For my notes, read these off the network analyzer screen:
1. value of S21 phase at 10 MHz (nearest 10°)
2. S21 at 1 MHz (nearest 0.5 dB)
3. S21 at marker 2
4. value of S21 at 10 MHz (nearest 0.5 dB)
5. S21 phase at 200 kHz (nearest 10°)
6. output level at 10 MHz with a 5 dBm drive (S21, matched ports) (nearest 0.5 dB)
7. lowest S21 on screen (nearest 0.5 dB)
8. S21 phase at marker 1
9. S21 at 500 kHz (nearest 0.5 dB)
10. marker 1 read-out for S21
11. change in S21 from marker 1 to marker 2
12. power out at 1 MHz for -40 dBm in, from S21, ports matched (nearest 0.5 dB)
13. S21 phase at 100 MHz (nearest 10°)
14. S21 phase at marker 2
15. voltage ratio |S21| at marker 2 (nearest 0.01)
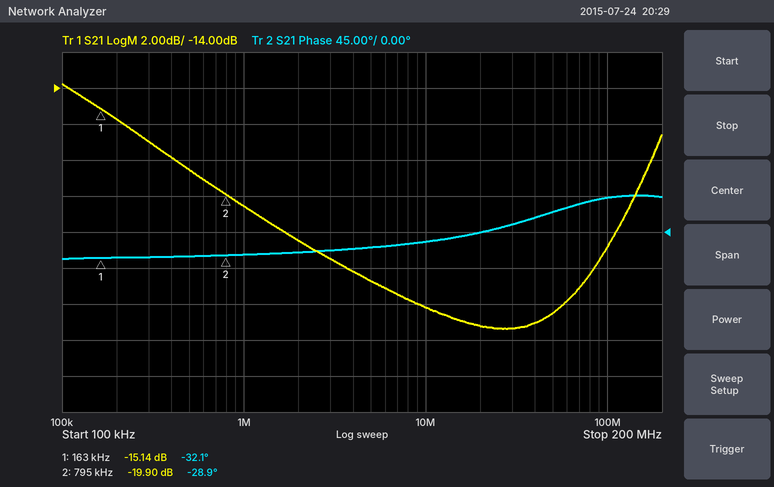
-10°
-20.5 dB
-19.90 dB
-26.0 dB
-30°
-21.0 dBm
-27.5 dB
-32.1°
-18.5 dB
-15.14 dB
-4.76 dB
-60.5 dBm
40°
-28.9°
0.10
